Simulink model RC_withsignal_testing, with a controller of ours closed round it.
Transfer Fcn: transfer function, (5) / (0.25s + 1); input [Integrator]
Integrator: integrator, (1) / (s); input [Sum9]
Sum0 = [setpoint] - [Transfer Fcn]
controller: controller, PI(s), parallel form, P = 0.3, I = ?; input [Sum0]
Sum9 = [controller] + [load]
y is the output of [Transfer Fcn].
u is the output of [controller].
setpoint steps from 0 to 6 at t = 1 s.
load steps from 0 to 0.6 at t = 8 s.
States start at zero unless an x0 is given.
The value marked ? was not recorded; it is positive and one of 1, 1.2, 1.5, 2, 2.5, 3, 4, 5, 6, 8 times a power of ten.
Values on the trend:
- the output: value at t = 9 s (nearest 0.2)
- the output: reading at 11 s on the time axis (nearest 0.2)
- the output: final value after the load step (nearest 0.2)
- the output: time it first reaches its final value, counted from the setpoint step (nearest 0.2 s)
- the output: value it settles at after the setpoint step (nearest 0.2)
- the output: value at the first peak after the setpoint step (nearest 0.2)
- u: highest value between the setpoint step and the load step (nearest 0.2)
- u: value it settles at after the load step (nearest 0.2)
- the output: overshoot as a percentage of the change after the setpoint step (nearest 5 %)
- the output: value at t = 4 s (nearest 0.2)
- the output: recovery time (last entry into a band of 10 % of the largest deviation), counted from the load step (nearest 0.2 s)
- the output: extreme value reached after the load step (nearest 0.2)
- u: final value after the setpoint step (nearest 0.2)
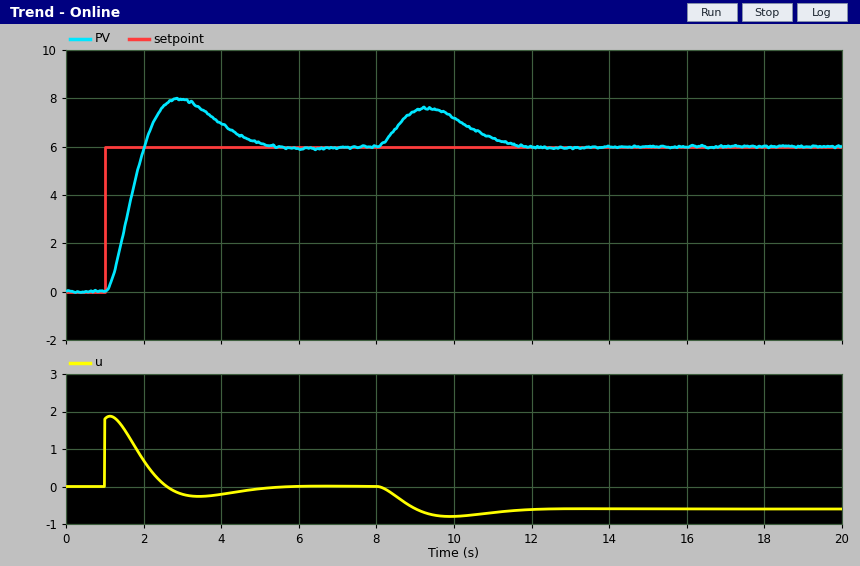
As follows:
7.4
6.4
6.0
1.0 s
6.0
8.0
1.8
-0.6
35 %
7.0
3.4 s
7.6
0.0
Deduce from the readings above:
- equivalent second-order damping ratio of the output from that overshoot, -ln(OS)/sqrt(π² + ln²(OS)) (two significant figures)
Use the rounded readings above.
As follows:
0.32
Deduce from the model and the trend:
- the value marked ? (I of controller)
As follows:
0.2
